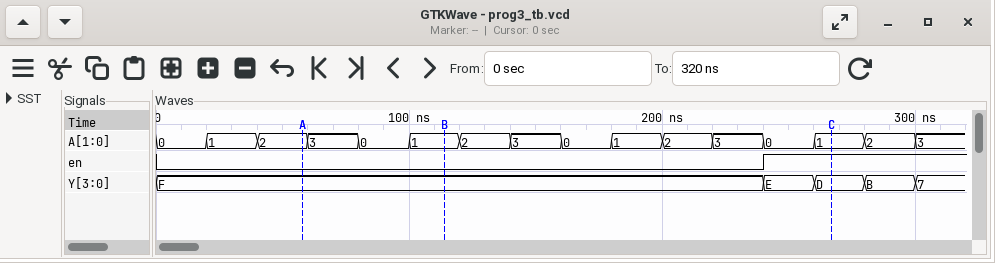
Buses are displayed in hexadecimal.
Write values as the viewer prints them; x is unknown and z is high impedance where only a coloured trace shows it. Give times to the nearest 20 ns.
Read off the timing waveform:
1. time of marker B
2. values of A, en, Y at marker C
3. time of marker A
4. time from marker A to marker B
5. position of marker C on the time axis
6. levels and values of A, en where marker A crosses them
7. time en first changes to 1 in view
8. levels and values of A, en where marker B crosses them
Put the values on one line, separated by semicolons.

120 ns; A=1, en=1, Y=D; 60 ns; 60 ns; 260 ns; A=2, en=0; 240 ns; A=1, en=0
